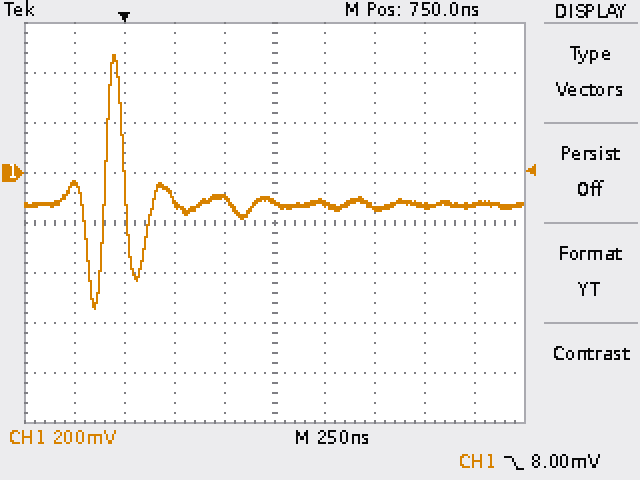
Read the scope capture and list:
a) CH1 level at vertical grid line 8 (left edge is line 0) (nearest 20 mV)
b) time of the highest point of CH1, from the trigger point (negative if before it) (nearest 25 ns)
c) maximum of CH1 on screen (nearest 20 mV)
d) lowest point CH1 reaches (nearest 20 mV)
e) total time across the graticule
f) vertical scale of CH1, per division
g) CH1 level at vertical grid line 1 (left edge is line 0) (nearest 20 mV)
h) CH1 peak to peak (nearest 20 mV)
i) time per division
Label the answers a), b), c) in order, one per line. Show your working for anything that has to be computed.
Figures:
a) -140 mV
b) -50 ns
c) 480 mV
d) -540 mV
e) 2.5 µs
f) 200 mV
g) -40 mV
h) 480 mV − (-540 mV) = 1.02 V
i) 250 ns
